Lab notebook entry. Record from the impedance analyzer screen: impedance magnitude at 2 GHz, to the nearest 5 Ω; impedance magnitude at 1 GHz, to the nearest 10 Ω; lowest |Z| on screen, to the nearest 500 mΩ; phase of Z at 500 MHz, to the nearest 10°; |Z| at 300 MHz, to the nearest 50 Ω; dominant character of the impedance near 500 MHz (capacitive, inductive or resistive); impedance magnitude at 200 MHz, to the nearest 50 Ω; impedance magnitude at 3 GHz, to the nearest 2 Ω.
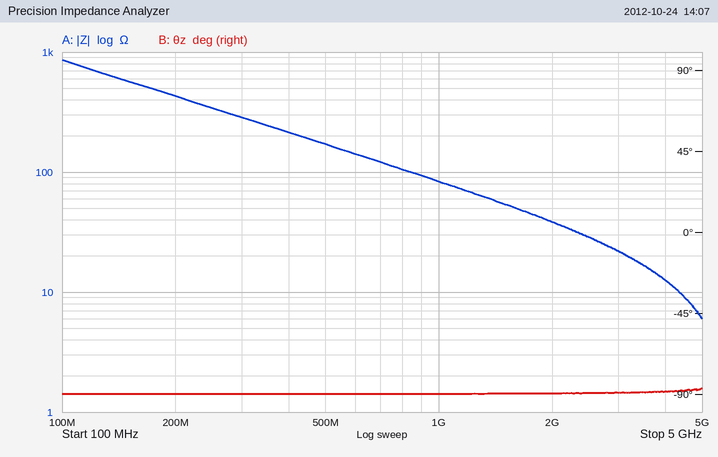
40 Ω
80 Ω
6.0 Ω
-90°
300 Ω
capacitive
450 Ω
22 Ω
